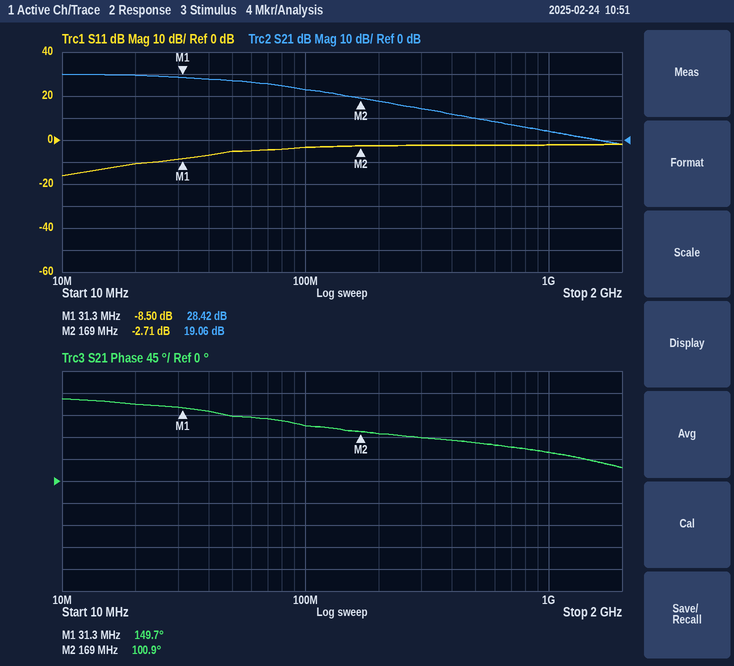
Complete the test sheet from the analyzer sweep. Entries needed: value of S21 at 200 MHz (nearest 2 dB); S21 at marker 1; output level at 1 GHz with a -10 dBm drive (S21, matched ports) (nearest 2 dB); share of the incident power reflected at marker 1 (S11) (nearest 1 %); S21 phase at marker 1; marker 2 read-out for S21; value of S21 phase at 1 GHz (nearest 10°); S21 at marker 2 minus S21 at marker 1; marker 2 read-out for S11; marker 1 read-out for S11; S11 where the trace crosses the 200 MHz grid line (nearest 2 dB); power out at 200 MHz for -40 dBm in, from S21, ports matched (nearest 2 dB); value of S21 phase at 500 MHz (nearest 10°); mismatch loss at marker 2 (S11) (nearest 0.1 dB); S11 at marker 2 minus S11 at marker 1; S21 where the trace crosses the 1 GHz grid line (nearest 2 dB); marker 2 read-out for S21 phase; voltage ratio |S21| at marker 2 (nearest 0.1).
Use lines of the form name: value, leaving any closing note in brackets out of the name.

value of S21 at 200 MHz: 18 dB
S21 at marker 1: 28.42 dB
output level at 1 GHz with a -10 dBm drive (S21, matched ports): -6 dBm
share of the incident power reflected at marker 1 (S11): 14 %
S21 phase at marker 1: 149.7°
marker 2 read-out for S21: 19.06 dB
value of S21 phase at 1 GHz: 60°
S21 at marker 2 minus S21 at marker 1: -9.36 dB
marker 2 read-out for S11: -2.71 dB
marker 1 read-out for S11: -8.50 dB
S11 where the trace crosses the 200 MHz grid line: -2 dB
power out at 200 MHz for -40 dBm in, from S21, ports matched: -22 dBm
value of S21 phase at 500 MHz: 80°
mismatch loss at marker 2 (S11): 3.3 dB
S11 at marker 2 minus S11 at marker 1: 5.79 dB
S21 where the trace crosses the 1 GHz grid line: 4 dB
marker 2 read-out for S21 phase: 100.9°
voltage ratio |S21| at marker 2: 9.0
